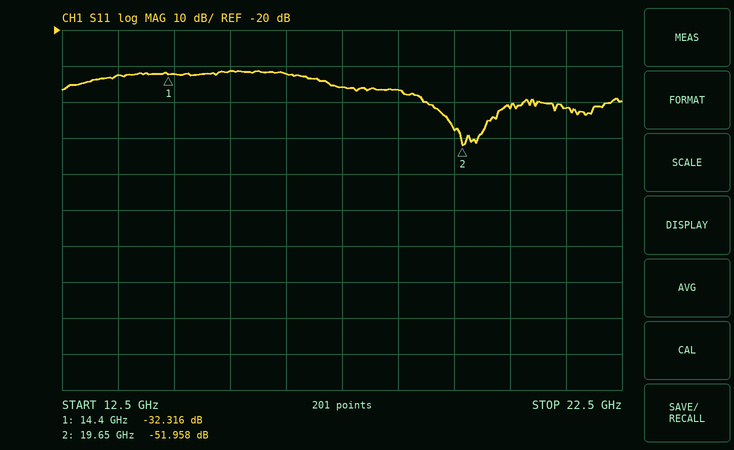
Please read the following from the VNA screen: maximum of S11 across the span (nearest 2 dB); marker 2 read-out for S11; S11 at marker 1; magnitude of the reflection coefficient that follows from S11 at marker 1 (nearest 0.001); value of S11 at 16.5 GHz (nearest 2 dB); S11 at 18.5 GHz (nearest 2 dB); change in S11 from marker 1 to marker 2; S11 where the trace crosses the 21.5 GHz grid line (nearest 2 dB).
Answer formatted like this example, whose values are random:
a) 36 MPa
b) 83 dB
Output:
a) -32 dB
b) -51.958 dB
c) -32.316 dB
d) 0.024
e) -32 dB
f) -36 dB
g) -19.642 dB
h) -42 dB
